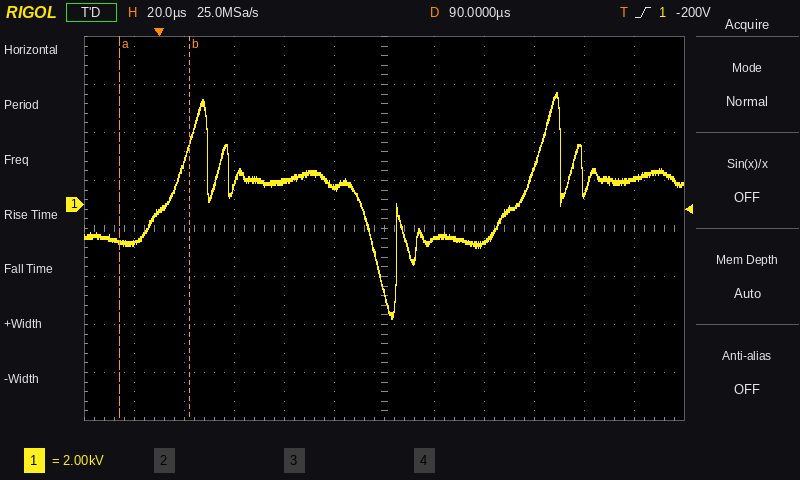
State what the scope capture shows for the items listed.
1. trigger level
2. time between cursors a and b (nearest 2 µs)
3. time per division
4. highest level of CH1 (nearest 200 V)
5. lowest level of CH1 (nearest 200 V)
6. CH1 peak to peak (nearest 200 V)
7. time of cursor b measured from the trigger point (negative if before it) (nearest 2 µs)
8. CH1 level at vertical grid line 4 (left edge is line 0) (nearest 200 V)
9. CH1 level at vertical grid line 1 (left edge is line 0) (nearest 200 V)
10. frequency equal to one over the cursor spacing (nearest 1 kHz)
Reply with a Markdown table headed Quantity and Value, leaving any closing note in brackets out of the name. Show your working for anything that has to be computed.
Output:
| Quantity | Value |
|---|---|
| trigger level | -200 V |
| time between cursors a and b | 28 µs |
| time per division | 20 µs |
| highest level of CH1 | 4.6 kV |
| lowest level of CH1 | -4.8 kV |
| CH1 peak to peak | 4.6 kV − (-4.8 kV) = 9.4 kV |
| time of cursor b measured from the trigger point (negative if before it) | +12 µs |
| CH1 level at vertical grid line 4 (left edge is line 0) | 1.0 kV |
| CH1 level at vertical grid line 1 (left edge is line 0) | -1.6 kV |
| frequency equal to one over the cursor spacing | 1 / 28 µs ≈ 36 kHz |
